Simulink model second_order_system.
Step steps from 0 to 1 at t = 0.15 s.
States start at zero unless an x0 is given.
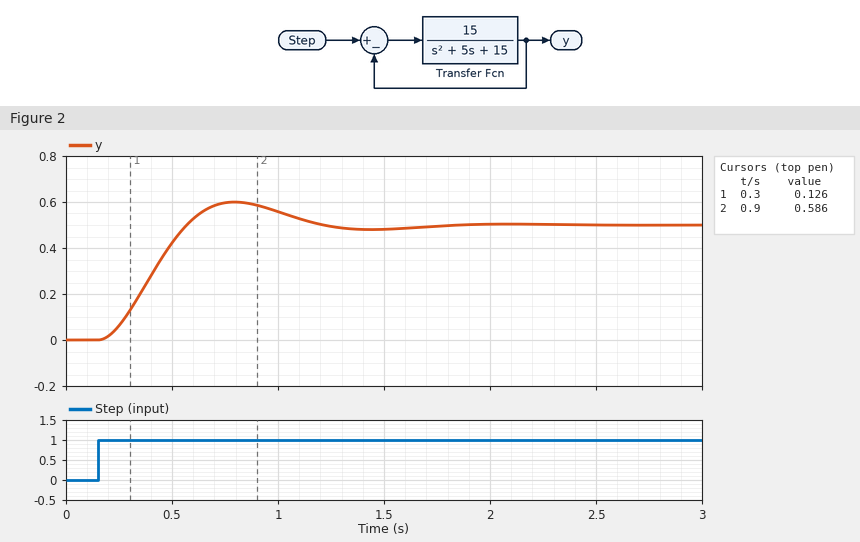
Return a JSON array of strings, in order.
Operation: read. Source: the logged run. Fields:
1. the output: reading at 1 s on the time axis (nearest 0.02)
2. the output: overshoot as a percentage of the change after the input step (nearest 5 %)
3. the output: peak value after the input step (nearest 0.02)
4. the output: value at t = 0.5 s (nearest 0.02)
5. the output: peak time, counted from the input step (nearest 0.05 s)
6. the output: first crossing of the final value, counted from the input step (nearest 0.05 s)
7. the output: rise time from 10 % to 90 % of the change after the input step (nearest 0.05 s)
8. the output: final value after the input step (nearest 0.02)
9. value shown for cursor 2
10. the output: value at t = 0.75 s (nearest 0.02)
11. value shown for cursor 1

["0.56", "20 %", "0.60", "0.42", "0.65 s", "0.40 s", "0.30 s", "0.50", "0.586", "0.60", "0.126"]
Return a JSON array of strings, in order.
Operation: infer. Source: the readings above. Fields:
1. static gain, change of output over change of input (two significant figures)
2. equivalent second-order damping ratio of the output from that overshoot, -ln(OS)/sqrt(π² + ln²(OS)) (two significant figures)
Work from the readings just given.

["0.50", "0.46"]
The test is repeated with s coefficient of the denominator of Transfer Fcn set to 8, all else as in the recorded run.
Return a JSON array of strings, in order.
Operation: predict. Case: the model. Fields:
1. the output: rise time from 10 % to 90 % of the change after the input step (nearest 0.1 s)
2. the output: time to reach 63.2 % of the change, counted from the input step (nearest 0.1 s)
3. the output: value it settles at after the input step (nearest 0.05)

["0.4 s", "0.3 s", "0.50"]
